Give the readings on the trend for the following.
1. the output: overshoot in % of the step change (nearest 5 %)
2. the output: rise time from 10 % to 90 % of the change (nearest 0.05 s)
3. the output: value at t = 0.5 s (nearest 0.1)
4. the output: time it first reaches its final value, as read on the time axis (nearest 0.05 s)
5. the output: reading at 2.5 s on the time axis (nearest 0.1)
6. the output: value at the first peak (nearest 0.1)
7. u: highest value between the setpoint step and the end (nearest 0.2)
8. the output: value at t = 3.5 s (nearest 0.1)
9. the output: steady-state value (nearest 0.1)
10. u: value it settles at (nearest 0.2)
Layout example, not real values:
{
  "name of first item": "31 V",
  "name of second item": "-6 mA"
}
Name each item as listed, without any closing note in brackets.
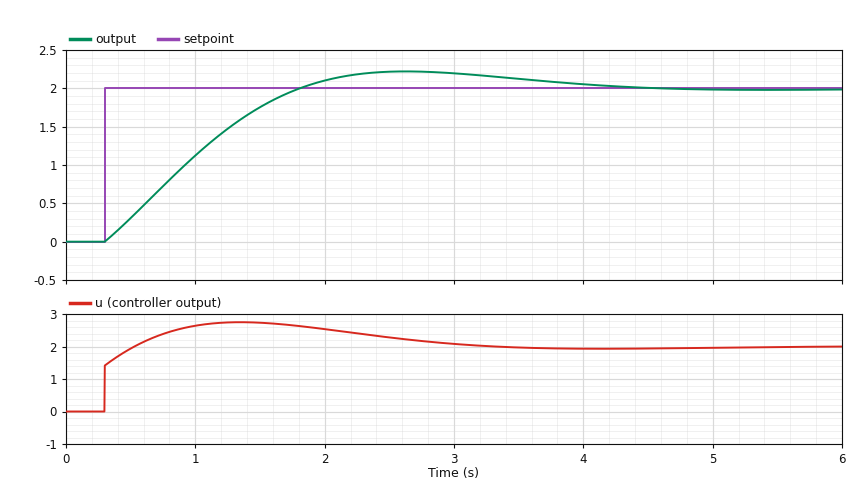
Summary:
{
  "the output: overshoot in % of the step change": "10 %",
  "the output: rise time from 10 % to 90 % of the change": "1.10 s",
  "the output: value at t = 0.5 s": "0.3",
  "the output: time it first reaches its final value, as read on the time axis": "1.80 s",
  "the output: reading at 2.5 s on the time axis": "2.2",
  "the output: value at the first peak": "2.2",
  "u: highest value between the setpoint step and the end": "2.8",
  "the output: value at t = 3.5 s": "2.1",
  "the output: steady-state value": "2.0",
  "u: value it settles at": "2.0"
}
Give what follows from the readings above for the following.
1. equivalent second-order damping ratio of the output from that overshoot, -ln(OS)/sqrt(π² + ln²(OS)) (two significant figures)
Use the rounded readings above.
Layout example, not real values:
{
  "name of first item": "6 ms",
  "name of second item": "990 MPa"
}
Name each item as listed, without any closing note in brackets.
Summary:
{
  "equivalent second-order damping ratio of the output from that overshoot, -ln(OS)/sqrt(π² + ln²(OS))": "0.59"
}
